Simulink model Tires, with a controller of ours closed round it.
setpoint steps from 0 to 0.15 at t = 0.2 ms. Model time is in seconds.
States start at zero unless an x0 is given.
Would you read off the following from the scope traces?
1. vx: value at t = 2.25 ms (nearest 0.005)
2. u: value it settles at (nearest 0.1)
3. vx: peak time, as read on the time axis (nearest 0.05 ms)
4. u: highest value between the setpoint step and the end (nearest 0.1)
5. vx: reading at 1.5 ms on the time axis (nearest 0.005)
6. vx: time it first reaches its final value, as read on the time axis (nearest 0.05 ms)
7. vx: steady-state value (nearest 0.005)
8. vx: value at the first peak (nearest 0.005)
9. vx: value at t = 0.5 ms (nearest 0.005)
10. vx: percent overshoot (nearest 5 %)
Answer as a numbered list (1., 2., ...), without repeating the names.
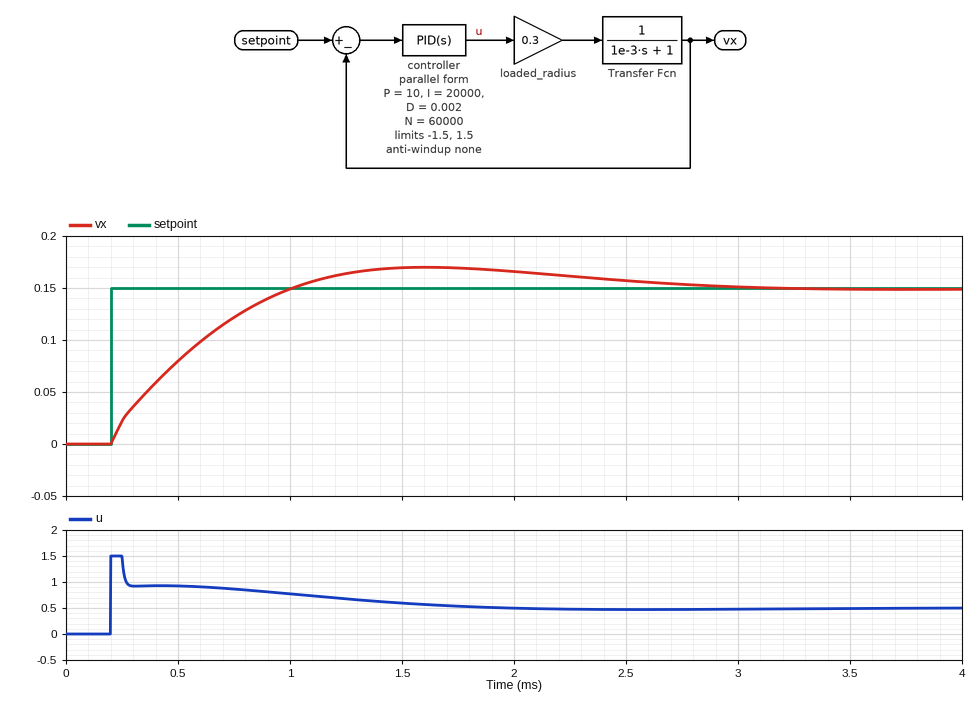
1. 0.160
2. 0.5
3. 1.60 ms
4. 1.5
5. 0.170
6. 1.00 ms
7. 0.150
8. 0.170
9. 0.080
10. 15 %
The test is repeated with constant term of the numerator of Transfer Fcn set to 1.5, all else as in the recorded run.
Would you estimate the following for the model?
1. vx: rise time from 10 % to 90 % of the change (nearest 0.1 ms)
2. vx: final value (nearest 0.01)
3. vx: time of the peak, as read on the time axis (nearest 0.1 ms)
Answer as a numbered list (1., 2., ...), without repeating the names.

1. 0.5 ms
2. 0.15
3. 1.4 ms
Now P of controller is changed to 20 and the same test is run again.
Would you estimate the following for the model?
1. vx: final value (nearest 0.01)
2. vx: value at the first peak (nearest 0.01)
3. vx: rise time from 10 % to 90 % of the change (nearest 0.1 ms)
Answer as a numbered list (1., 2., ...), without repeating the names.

1. 0.15
2. 0.16
3. 0.5 ms
